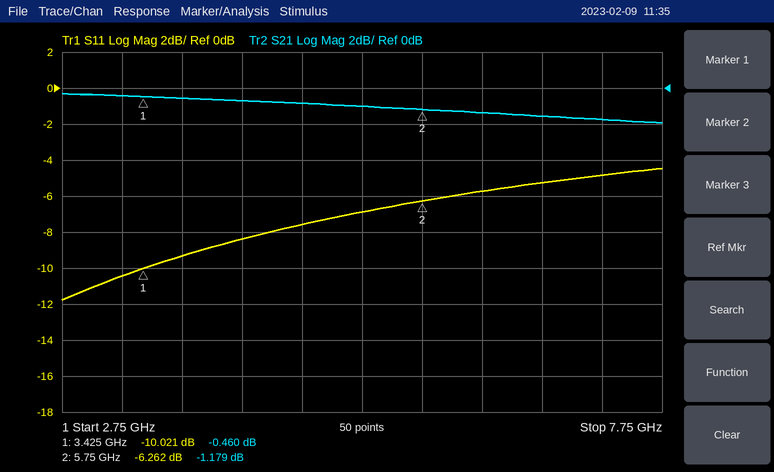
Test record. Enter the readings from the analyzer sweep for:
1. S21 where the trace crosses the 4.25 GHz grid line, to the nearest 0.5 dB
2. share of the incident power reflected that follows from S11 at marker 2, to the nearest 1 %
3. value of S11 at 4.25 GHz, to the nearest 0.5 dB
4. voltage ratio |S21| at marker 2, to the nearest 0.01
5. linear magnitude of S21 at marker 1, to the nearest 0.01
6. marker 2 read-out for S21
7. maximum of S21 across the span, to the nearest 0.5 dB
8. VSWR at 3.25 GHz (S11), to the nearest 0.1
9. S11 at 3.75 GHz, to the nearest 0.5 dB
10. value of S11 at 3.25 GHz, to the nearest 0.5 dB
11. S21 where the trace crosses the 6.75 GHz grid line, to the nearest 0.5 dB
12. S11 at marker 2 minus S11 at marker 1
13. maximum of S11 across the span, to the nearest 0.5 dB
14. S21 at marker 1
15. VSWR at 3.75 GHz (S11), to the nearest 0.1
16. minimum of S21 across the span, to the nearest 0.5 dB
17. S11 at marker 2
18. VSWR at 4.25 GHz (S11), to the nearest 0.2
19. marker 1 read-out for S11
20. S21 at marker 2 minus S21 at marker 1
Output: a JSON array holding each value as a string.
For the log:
["-0.5 dB", "24 %", "-8.5 dB", "0.87", "0.95", "-1.179 dB", "-0.5 dB", "1.9", "-9.5 dB", "-10.5 dB", "-1.5 dB", "3.759 dB", "-4.5 dB", "-0.460 dB", "2.0", "-2.0 dB", "-6.262 dB", "2.2", "-10.021 dB", "-0.719 dB"]
